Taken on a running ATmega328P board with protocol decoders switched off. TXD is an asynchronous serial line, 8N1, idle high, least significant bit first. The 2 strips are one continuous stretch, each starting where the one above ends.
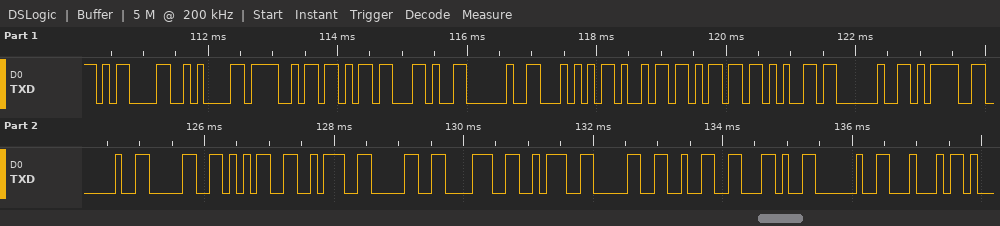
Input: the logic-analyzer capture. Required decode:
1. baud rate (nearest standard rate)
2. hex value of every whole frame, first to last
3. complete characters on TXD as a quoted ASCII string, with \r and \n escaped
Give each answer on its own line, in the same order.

9600 baud
0x0D 0x0A 0x4F 0x6B 0x2C 0x20 0x54 0x69 0x6D 0x65 0x20 0x3D 0x20 0x30 0x35 0x3A 0x30 0x38 0x3A 0x30 0x32 0x2C 0x20 0x44
"\r\nOk, Time = 05:08:02, D"
